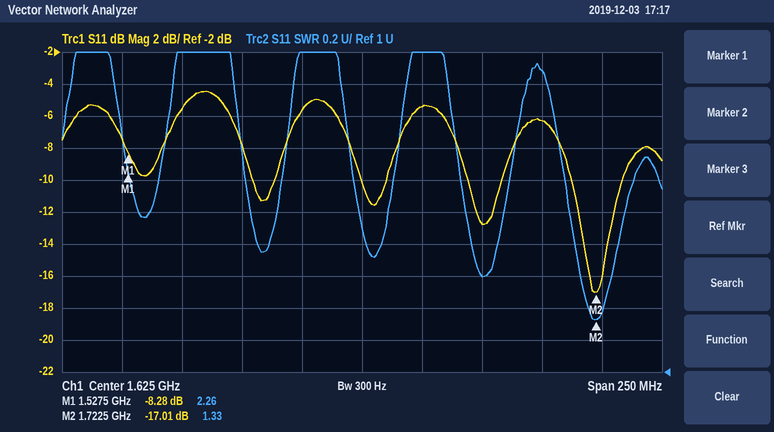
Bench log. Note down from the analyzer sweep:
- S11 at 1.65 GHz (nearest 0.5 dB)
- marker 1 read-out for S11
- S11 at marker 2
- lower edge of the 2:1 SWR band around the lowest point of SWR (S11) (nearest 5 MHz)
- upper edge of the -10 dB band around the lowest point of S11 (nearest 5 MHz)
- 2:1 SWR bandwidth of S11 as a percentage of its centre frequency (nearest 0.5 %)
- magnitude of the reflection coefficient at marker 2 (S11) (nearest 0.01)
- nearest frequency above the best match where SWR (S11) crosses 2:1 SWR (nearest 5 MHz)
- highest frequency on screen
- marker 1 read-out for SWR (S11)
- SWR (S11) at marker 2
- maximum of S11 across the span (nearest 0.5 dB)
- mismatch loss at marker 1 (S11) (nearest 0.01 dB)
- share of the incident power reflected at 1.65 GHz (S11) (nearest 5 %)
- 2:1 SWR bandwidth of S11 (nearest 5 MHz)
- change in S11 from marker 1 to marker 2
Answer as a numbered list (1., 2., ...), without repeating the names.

1. -5.5 dB
2. -8.28 dB
3. -17.01 dB
4. 1.710 GHz
5. 1.735 GHz
6. 1.5 %
7. 0.14
8. 1.735 GHz
9. 1.75 GHz
10. 2.26
11. 1.33
12. -4.5 dB
13. 0.70 dB
14. 30 %
15. 25 MHz
16. -8.73 dB
